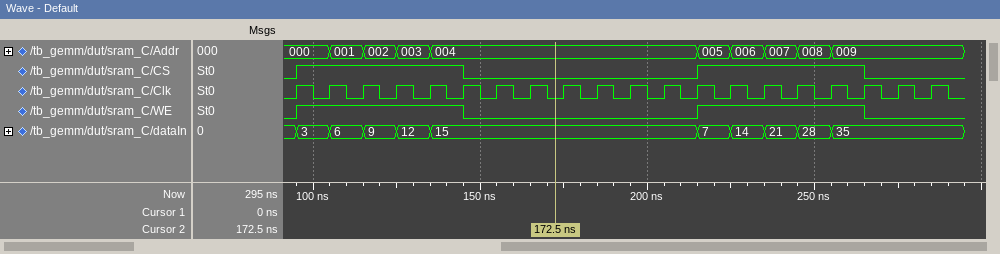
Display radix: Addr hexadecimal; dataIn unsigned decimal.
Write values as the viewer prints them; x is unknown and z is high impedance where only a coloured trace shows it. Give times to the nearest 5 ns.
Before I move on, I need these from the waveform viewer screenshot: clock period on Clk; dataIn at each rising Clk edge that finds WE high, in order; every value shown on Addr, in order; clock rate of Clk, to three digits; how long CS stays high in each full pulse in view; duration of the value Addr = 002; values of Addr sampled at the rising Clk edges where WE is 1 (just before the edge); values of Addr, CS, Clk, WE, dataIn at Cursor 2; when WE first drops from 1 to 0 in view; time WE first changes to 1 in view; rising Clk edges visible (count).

10 ns
3, 6, 9, 12, 15, 7, 14, 21, 28, 35
000, 001, 002, 003, 004, 005, 006, 007, 008, 009
100 MHz
50 ns, 50 ns
10 ns
000, 001, 002, 003, 004, 005, 006, 007, 008, 009
Addr=004, CS=0, Clk=0, WE=0, dataIn=15
145 ns
95 ns
20
